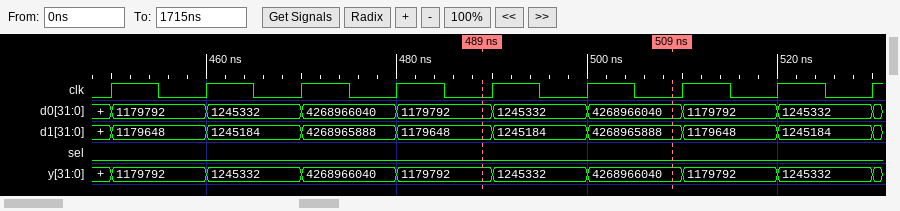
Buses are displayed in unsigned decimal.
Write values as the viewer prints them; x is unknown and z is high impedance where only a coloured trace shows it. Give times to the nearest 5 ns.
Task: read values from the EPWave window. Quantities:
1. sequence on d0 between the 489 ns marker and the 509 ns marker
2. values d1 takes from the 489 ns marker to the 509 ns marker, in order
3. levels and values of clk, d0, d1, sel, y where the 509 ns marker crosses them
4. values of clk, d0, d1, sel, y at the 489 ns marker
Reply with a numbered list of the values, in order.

1. 1179792, 1245332, 4268966040
2. 1179648, 1245184, 4268965888
3. clk=0, d0=4268966040, d1=4268965888, sel=0, y=4268966040
4. clk=0, d0=1179792, d1=1179648, sel=0, y=1179792
